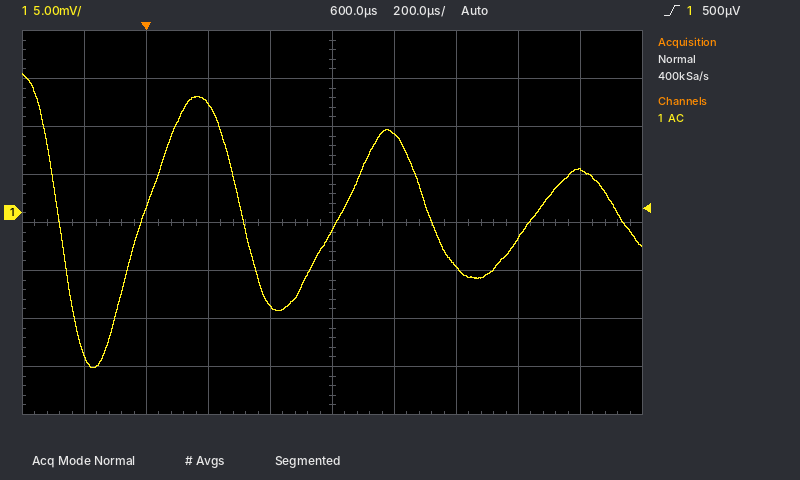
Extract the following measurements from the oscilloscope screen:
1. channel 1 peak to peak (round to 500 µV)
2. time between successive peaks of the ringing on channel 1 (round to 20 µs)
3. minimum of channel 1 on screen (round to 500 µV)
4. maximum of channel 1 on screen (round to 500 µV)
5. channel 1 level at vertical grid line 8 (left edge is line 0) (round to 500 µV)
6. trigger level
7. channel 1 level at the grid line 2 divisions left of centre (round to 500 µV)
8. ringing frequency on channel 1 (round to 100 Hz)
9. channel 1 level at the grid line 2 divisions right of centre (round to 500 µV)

30.5 mV
620 µs
-16.0 mV
14.5 mV
-2.5 mV
500 µV
11.5 mV
1.6 kHz
-5.5 mV
